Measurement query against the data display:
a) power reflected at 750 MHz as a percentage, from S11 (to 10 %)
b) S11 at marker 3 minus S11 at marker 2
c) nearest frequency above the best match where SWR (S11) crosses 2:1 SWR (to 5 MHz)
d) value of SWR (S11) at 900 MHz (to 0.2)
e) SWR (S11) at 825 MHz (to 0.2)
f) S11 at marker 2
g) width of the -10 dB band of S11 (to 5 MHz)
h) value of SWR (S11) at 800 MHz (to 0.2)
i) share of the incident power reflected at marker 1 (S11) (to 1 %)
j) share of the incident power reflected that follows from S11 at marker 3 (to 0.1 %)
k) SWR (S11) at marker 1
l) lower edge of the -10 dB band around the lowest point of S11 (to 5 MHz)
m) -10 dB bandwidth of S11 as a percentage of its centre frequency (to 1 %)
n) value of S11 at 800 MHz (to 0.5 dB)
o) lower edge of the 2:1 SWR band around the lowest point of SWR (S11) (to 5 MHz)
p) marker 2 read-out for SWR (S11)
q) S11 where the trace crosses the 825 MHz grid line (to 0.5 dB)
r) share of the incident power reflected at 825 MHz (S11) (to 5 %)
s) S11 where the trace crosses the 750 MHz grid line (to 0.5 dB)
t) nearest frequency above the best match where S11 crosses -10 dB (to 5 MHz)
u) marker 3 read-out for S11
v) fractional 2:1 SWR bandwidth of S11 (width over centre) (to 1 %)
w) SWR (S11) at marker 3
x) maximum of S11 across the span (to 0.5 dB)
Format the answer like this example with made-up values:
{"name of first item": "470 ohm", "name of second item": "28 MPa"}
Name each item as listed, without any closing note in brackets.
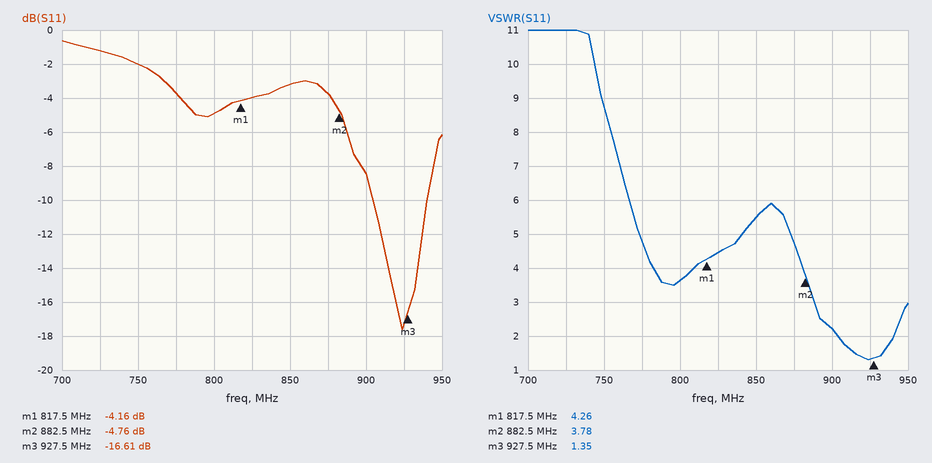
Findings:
{"power reflected at 750 MHz as a percentage, from S11": "60 %", "S11 at marker 3 minus S11 at marker 2": "-11.85 dB", "nearest frequency above the best match where SWR (S11) crosses 2:1 SWR": "940 MHz", "value of SWR (S11) at 900 MHz": "2.2", "SWR (S11) at 825 MHz": "4.4", "S11 at marker 2": "-4.76 dB", "width of the -10 dB band of S11": "35 MHz", "value of SWR (S11) at 800 MHz": "3.6", "share of the incident power reflected at marker 1 (S11)": "38 %", "share of the incident power reflected that follows from S11 at marker 3": "2.2 %", "SWR (S11) at marker 1": "4.26", "lower edge of the -10 dB band around the lowest point of S11": "905 MHz", "-10 dB bandwidth of S11 as a percentage of its centre frequency": "4 %", "value of S11 at 800 MHz": "-5.0 dB", "lower edge of the 2:1 SWR band around the lowest point of SWR (S11)": "905 MHz", "marker 2 read-out for SWR": "3.78", "S11 where the trace crosses the 825 MHz grid line": "-4.0 dB", "share of the incident power reflected at 825 MHz (S11)": "40 %", "S11 where the trace crosses the 750 MHz grid line": "-2.0 dB", "nearest frequency above the best match where S11 crosses -10 dB": "940 MHz", "marker 3 read-out for S11": "-16.61 dB", "fractional 2:1 SWR bandwidth of S11 (width over centre)": "4 %", "SWR (S11) at marker 3": "1.35", "maximum of S11 across the span": "-0.5 dB"}
